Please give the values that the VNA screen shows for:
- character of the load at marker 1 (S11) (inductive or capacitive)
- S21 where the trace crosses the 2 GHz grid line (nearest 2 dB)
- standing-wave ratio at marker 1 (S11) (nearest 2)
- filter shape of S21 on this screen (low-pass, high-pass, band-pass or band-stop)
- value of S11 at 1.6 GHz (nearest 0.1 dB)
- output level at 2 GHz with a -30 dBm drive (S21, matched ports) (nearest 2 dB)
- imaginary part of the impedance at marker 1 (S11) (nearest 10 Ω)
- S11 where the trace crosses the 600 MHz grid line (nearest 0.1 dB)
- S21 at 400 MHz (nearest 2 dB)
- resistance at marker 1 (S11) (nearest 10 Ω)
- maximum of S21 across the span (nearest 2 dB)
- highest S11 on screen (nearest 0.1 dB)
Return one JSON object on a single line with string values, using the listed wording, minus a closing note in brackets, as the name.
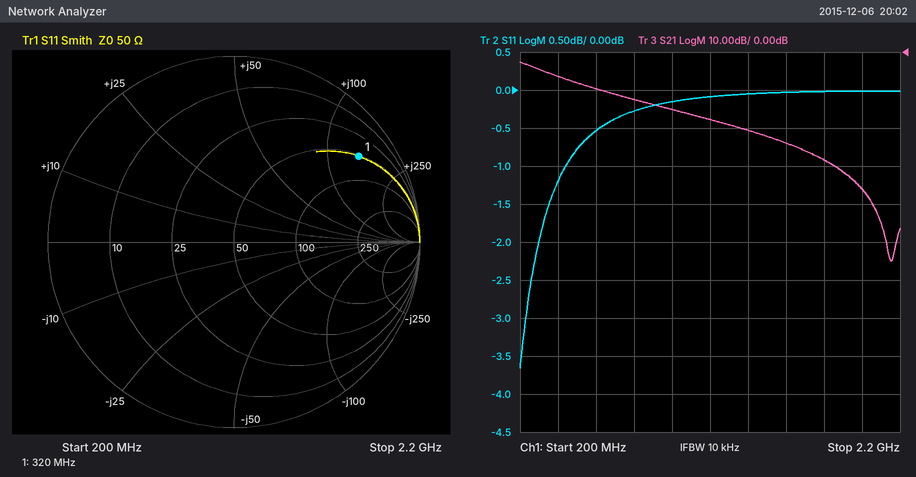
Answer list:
{"character of the load at marker 1 (S11)": "inductive", "S21 where the trace crosses the 2 GHz grid line": "-36 dB", "standing-wave ratio at marker 1 (S11)": "10", "filter shape of S21 on this screen": "low-pass", "value of S11 at 1.6 GHz": "0.0 dB", "output level at 2 GHz with a -30 dBm drive (S21, matched ports)": "-66 dBm", "imaginary part of the impedance at marker 1 (S11)": "+140 Ω", "S11 where the trace crosses the 600 MHz grid line": "-0.5 dB", "S21 at 400 MHz": "-6 dB", "resistance at marker 1 (S11)": "50 Ω", "maximum of S21 across the span": "-2 dB", "highest S11 on screen": "0.0 dB"}
